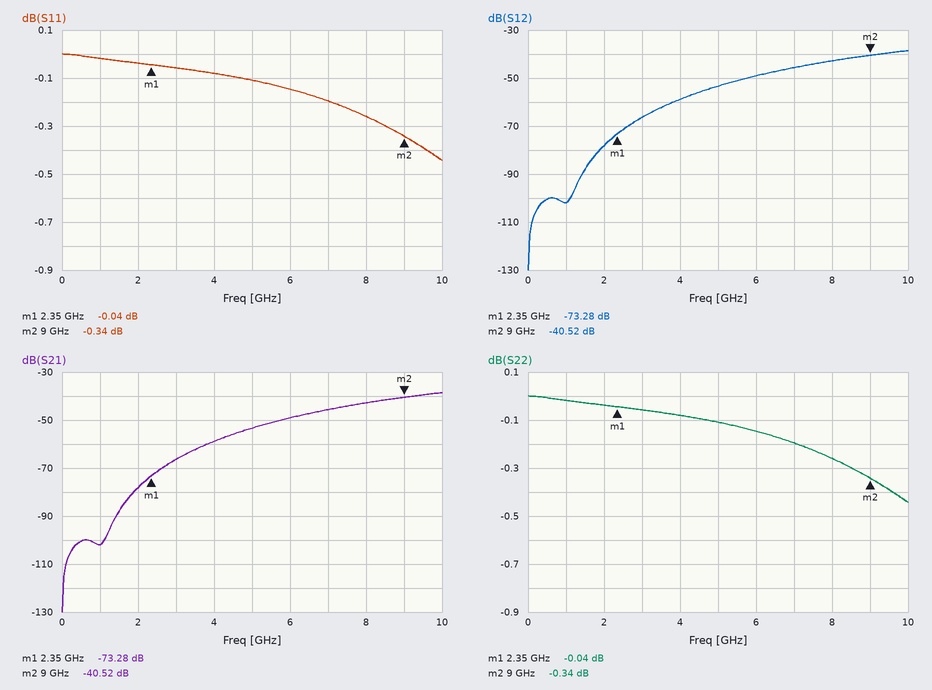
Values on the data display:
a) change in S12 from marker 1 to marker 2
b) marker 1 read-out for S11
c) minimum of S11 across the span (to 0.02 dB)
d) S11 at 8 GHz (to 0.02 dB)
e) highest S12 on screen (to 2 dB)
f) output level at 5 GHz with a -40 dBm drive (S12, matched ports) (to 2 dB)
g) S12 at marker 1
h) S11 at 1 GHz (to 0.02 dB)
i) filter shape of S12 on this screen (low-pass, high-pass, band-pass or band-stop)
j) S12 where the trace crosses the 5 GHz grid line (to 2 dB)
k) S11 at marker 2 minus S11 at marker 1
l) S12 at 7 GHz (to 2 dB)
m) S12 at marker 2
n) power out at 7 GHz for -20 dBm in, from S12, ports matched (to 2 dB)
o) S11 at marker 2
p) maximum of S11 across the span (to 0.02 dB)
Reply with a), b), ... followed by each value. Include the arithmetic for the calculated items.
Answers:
a) -40.52 − (-73.28) = 32.76 dB
b) -0.04 dB
c) -0.44 dB
d) -0.26 dB
e) -38 dB
f) -40 dBm + (-54 dB) = -94 dBm
g) -73.28 dB
h) -0.02 dB
i) high-pass
j) -54 dB
k) -0.34 − (-0.04) = -0.30 dB
l) -46 dB
m) -40.52 dB
n) -20 dBm + (-46 dB) = -66 dBm
o) -0.34 dB
p) 0.00 dB
